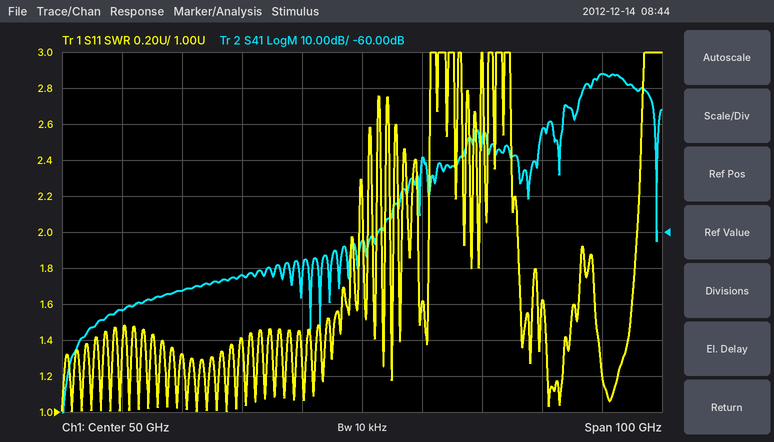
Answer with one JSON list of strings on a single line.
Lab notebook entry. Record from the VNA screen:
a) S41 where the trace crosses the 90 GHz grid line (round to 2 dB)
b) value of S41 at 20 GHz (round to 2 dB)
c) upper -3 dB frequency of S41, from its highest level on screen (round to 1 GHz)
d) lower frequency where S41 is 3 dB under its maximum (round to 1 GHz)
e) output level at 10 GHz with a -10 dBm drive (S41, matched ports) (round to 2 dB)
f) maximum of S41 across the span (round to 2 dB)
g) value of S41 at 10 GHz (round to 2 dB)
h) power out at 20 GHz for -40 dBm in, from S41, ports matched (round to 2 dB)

["-16 dB", "-76 dB", "94 GHz", "88 GHz", "-92 dBm", "-16 dB", "-82 dB", "-116 dBm"]
